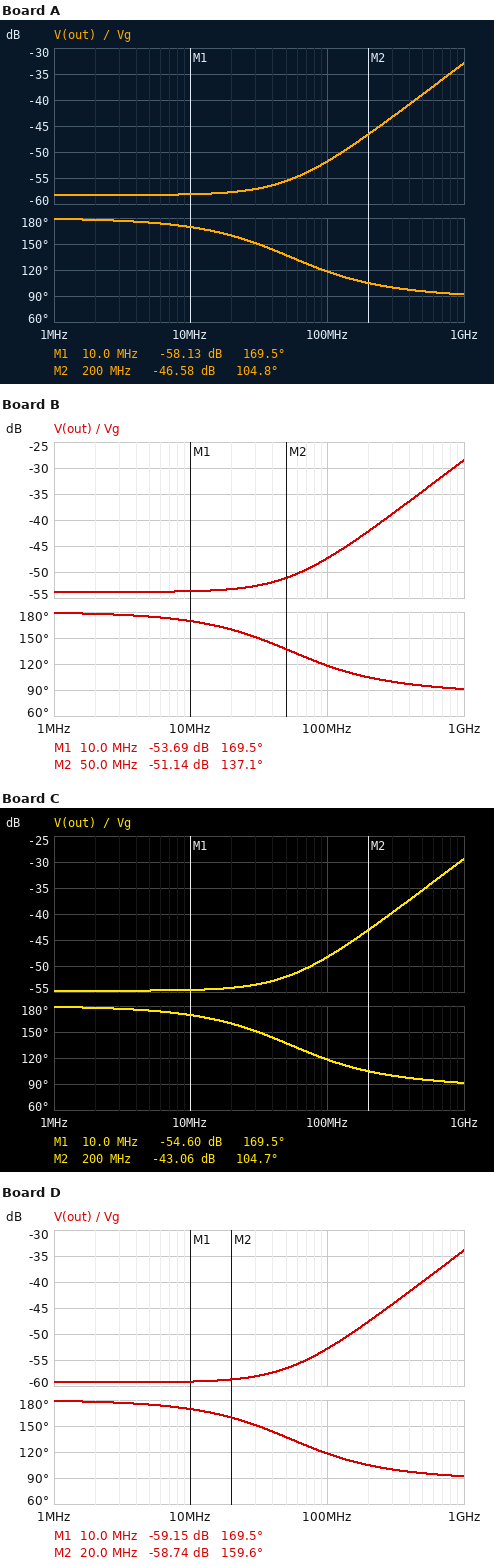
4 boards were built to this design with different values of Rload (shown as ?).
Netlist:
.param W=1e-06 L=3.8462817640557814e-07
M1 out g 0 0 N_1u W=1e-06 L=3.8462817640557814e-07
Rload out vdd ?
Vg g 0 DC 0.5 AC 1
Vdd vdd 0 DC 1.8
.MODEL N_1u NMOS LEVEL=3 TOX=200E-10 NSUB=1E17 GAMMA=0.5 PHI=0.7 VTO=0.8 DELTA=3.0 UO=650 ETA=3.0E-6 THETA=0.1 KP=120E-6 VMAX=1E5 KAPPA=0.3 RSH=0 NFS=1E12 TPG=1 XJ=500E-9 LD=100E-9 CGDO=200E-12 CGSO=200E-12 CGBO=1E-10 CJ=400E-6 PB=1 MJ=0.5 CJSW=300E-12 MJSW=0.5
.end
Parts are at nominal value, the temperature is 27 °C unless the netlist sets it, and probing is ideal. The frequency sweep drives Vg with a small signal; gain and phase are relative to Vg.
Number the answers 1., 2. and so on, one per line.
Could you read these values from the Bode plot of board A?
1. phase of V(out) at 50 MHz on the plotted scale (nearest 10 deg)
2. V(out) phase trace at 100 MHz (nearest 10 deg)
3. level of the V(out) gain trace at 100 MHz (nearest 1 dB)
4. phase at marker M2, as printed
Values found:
1. 140 deg
2. 120 deg
3. -52 dB
4. 104.8 deg
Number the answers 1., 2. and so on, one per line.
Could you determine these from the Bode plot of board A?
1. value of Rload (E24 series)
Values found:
1. 18 kΩ
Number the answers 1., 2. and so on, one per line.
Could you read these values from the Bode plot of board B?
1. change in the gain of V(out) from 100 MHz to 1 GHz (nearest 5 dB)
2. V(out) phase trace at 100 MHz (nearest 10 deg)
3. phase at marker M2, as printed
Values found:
1. 20 dB
2. 120 deg
3. 137.1 deg
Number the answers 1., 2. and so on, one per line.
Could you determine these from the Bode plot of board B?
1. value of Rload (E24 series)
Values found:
1. 30 kΩ
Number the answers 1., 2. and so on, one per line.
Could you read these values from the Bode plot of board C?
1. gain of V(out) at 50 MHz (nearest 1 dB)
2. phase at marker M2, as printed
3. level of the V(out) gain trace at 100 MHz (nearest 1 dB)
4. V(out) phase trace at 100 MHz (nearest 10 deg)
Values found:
1. -52 dB
2. 104.7 deg
3. -48 dB
4. 120 deg
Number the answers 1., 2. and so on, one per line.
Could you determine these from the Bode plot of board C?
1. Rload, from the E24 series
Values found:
1. 27 kΩ
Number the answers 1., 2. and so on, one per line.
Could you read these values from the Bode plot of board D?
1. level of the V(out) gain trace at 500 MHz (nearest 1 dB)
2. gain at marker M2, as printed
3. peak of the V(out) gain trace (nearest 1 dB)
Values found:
1. -40 dB
2. -58.74 dB
3. -34 dB
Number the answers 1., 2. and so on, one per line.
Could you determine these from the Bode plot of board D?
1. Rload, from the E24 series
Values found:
1. 16 kΩ
